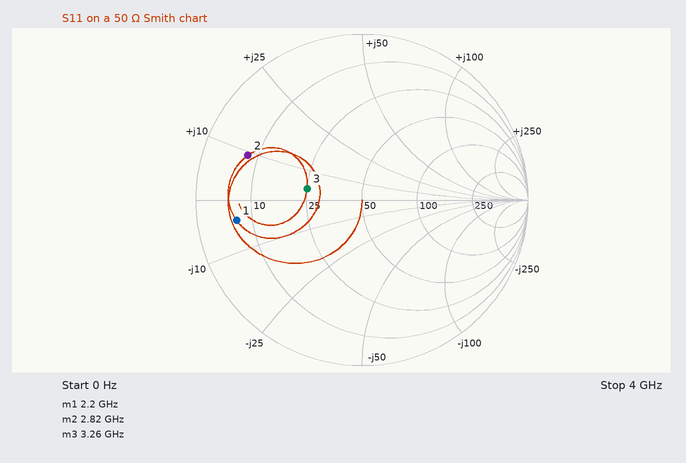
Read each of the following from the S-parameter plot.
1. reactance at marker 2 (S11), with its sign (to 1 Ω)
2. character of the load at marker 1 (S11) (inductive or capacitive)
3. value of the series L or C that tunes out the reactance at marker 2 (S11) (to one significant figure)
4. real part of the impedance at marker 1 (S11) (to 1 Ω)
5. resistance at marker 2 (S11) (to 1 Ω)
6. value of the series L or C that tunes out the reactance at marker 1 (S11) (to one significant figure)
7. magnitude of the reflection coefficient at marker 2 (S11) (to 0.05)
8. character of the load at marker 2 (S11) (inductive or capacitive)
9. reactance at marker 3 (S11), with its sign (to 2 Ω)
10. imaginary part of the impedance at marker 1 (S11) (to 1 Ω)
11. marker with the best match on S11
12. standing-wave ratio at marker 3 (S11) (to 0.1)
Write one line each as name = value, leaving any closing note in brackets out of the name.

reactance at marker 2 (S11), with its sign = +9 Ω
character of the load at marker 1 (S11) = capacitive
value of the series L or C that tunes out the reactance at marker 2 (S11) = 6 pF
real part of the impedance at marker 1 (S11) = 7 Ω
resistance at marker 2 (S11) = 8 Ω
value of the series L or C that tunes out the reactance at marker 1 (S11) = 300 pH
magnitude of the reflection coefficient at marker 2 (S11) = 0.75
character of the load at marker 2 (S11) = inductive
reactance at marker 3 (S11), with its sign = +4 Ω
imaginary part of the impedance at marker 1 (S11) = -4 Ω
marker with the best match on S11 = marker 3
standing-wave ratio at marker 3 (S11) = 2.0
